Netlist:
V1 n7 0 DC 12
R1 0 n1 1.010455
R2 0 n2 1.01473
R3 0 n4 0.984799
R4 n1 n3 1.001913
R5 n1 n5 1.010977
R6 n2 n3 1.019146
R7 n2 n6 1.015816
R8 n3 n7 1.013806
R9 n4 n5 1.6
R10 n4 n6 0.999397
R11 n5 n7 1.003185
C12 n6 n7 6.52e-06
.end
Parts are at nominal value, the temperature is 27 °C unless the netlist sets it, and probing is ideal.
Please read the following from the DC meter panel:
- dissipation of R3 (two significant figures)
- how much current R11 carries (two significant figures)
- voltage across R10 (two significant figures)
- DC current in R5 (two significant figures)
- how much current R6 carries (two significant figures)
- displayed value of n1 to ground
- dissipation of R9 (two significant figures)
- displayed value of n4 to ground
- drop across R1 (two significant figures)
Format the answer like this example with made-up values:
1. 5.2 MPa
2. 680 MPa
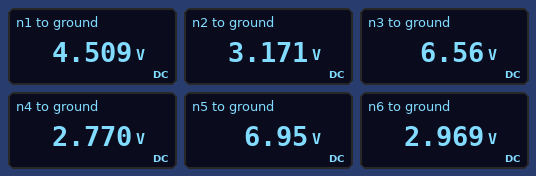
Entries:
1. 7.8 W
2. 5.0 A
3. 200 mV
4. 2.4 A
5. 3.3 A
6. 4.509 V
7. 11 W
8. 2.770 V
9. 4.5 V
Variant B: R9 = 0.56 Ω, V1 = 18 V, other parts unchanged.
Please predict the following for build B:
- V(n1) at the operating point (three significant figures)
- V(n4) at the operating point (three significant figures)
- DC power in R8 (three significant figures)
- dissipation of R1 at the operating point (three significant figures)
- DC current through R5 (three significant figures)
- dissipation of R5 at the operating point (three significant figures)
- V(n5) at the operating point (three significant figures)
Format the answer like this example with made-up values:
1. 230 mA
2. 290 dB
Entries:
1. 6.30 V
2. 5.69 V
3. 66.7 W
4. 39.3 W
5. 2.77 A
6. 7.76 W
7. 9.10 V
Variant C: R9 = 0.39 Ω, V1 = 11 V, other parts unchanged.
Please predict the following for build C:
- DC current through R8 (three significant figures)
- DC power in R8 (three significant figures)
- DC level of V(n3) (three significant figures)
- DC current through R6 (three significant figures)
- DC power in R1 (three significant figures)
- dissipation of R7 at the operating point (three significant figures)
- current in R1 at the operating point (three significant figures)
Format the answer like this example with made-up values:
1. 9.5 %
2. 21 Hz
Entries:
1. 4.97 A
2. 25.0 W
3. 5.96 V
4. 2.78 A
5. 14.1 W
6. 92.9 mW
7. 3.73 A
